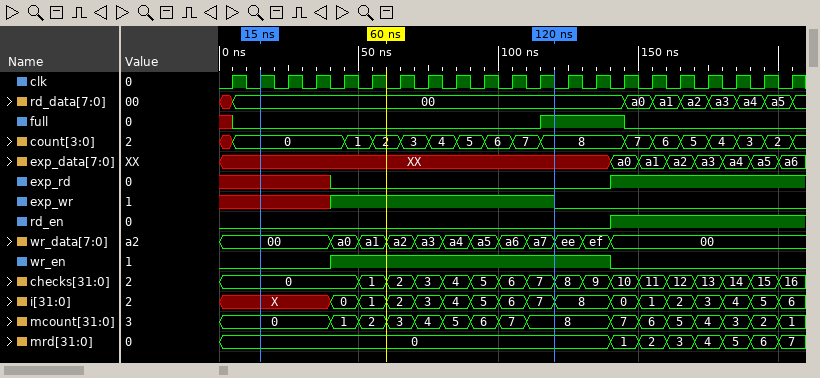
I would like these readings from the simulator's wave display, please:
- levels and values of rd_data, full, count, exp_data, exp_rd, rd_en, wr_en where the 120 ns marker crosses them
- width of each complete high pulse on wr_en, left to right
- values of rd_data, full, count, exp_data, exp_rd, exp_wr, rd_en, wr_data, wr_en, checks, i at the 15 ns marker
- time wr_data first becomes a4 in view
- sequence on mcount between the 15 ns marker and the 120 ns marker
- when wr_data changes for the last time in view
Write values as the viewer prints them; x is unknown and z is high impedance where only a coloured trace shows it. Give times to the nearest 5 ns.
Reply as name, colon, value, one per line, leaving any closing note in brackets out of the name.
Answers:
levels and values of rd_data, full, count, exp_data, exp_rd, rd_en, wr_en where the 120 ns marker crosses them: rd_data=00, full=1, count=8, exp_data=XX, exp_rd=0, rd_en=0, wr_en=1
width of each complete high pulse on wr_en, left to right: 100 ns
values of rd_data, full, count, exp_data, exp_rd, exp_wr, rd_en, wr_data, wr_en, checks, i at the 15 ns marker: rd_data=00, full=0, count=0, exp_data=XX, exp_rd=x, exp_wr=x, rd_en=0, wr_data=00, wr_en=0, checks=0, i=X
time wr_data first becomes a4 in view: 80 ns
sequence on mcount between the 15 ns marker and the 120 ns marker: 0, 1, 2, 3, 4, 5, 6, 7, 8
when wr_data changes for the last time in view: 140 ns
